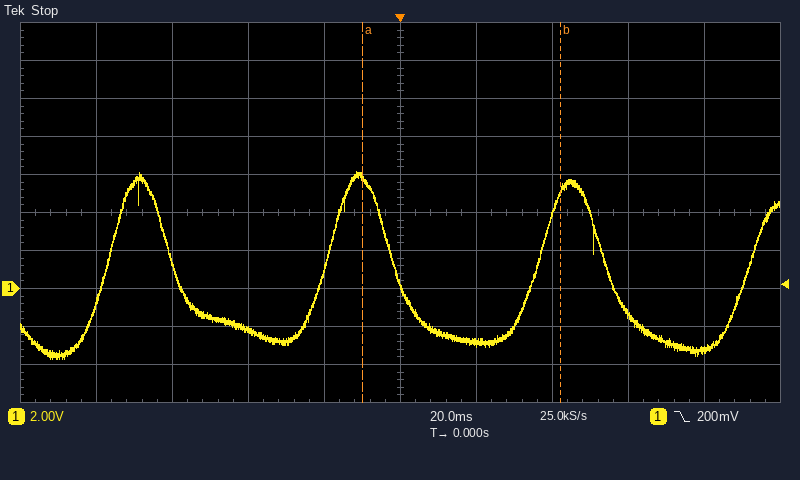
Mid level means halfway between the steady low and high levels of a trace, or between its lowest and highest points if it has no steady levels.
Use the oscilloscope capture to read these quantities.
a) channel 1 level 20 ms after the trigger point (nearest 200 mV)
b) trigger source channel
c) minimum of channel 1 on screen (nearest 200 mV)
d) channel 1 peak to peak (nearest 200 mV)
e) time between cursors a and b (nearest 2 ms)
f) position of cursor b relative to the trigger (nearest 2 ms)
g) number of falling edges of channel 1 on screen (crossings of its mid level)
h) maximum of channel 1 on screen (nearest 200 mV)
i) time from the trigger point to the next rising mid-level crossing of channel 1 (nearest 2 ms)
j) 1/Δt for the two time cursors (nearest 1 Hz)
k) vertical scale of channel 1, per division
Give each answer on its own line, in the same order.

-2.8 V
channel 1
-3.6 V
9.8 V
52 ms
+42 ms
3
6.2 V
36 ms
19 Hz
2 V
